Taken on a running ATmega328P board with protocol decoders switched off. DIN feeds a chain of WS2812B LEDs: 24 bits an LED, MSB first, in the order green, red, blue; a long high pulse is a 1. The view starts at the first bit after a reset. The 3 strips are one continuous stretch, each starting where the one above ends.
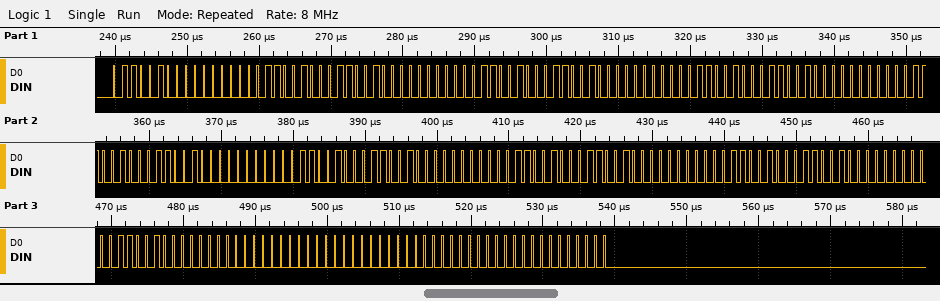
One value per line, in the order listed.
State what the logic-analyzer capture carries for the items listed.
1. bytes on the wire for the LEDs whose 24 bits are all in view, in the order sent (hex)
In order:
64 00 64 64 00 64 64 00 64 64 00 64 64 00 64 64 00 64 64 00 64 64 00 64 00 00 00 00 00 00
